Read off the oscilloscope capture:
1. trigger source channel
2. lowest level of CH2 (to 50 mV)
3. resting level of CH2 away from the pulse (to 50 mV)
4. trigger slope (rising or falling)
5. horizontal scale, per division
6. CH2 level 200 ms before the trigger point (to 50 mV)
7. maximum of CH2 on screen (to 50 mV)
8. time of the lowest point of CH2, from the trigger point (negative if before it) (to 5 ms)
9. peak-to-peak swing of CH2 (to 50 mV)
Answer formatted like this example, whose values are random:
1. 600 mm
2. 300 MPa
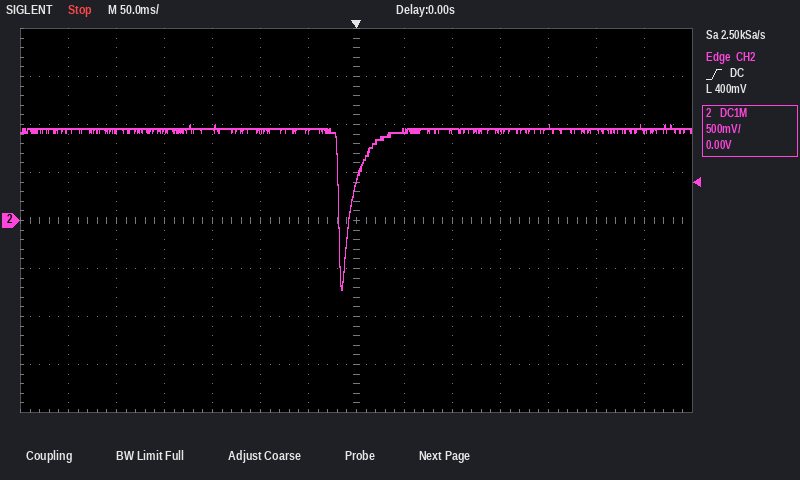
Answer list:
1. CH2
2. -700 mV
3. 950 mV
4. rising
5. 50 ms
6. 950 mV
7. 1.00 V
8. -15 ms
9. 1.70 V
